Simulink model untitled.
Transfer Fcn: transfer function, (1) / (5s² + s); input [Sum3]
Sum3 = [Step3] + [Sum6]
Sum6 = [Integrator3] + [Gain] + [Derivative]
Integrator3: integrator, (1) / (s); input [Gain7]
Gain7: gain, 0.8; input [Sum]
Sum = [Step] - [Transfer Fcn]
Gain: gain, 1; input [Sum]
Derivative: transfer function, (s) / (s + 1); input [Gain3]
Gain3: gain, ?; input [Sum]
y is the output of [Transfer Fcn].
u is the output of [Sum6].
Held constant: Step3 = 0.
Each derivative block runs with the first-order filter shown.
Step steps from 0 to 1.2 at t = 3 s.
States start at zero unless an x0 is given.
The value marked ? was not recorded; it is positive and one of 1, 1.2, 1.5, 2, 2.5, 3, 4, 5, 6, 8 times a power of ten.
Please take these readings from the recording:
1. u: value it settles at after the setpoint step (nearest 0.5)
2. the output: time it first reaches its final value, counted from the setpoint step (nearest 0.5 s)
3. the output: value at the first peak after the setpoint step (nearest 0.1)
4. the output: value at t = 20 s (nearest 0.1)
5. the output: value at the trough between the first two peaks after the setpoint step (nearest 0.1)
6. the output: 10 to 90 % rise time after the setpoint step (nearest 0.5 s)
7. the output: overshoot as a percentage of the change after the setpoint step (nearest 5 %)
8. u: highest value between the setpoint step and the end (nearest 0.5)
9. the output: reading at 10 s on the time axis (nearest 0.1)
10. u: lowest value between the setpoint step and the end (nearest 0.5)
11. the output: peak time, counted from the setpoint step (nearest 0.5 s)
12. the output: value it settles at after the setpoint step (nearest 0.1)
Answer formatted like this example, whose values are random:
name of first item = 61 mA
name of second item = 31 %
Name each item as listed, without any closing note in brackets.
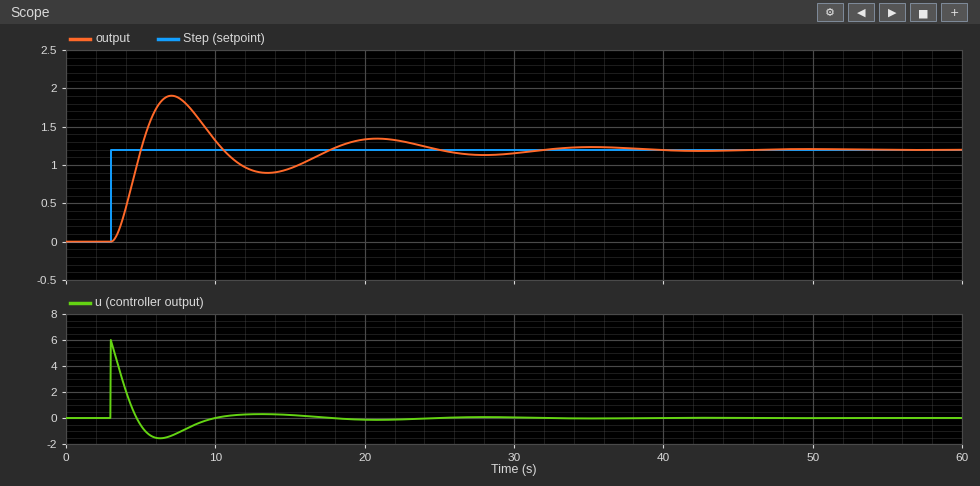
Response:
u: value it settles at after the setpoint step = 0.0
the output: time it first reaches its final value, counted from the setpoint step = 2.0 s
the output: value at the first peak after the setpoint step = 1.9
the output: value at t = 20 s = 1.3
the output: value at the trough between the first two peaks after the setpoint step = 0.9
the output: 10 to 90 % rise time after the setpoint step = 1.5 s
the output: overshoot as a percentage of the change after the setpoint step = 60 %
u: highest value between the setpoint step and the end = 6.0
the output: reading at 10 s on the time axis = 1.3
u: lowest value between the setpoint step and the end = -1.5
the output: peak time, counted from the setpoint step = 4.0 s
the output: value it settles at after the setpoint step = 1.2
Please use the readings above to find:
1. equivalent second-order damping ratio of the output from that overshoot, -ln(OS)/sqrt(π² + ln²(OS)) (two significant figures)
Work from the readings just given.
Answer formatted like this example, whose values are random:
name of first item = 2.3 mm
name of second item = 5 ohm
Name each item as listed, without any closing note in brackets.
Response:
equivalent second-order damping ratio of the output from that overshoot, -ln(OS)/sqrt(π² + ln²(OS)) = 0.16
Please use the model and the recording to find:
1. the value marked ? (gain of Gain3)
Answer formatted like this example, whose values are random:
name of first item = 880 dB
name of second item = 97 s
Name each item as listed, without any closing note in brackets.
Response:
the value marked ? = 4
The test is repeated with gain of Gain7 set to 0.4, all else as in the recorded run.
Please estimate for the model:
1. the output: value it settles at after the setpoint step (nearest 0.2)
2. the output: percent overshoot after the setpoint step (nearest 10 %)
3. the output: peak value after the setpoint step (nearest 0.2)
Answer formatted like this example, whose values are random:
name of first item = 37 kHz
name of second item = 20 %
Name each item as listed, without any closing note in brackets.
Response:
the output: value it settles at after the setpoint step = 1.2
the output: percent overshoot after the setpoint step = 40 %
the output: peak value after the setpoint step = 1.6
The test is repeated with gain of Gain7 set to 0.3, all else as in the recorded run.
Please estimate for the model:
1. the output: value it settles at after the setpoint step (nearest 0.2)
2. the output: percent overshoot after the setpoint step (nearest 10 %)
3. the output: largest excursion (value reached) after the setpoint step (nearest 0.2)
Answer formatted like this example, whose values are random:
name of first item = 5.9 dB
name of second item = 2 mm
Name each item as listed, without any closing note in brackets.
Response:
the output: value it settles at after the setpoint step = 1.2
the output: percent overshoot after the setpoint step = 30 %
the output: largest excursion (value reached) after the setpoint step = 1.6
